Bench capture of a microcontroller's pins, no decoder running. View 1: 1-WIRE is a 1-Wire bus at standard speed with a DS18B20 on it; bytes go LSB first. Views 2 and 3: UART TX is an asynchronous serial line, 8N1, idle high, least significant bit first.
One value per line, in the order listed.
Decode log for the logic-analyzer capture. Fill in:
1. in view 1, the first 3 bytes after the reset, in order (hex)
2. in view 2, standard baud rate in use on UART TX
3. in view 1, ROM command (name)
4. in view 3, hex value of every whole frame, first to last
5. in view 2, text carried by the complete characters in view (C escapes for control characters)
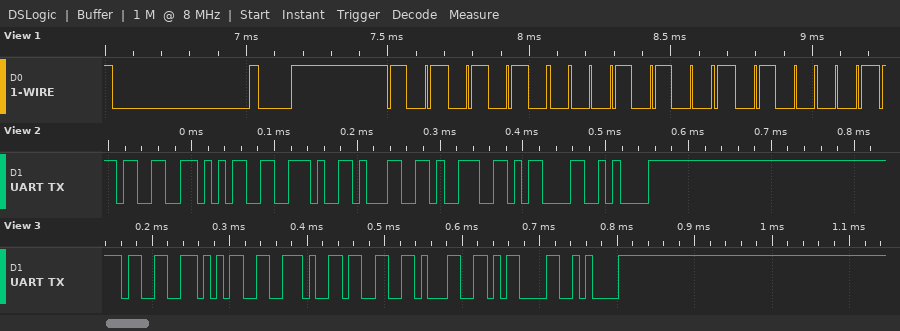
55 28 85
115200 baud
Match ROM
33 35 2E 33 31 0D 0A
"35.19\r\n"
